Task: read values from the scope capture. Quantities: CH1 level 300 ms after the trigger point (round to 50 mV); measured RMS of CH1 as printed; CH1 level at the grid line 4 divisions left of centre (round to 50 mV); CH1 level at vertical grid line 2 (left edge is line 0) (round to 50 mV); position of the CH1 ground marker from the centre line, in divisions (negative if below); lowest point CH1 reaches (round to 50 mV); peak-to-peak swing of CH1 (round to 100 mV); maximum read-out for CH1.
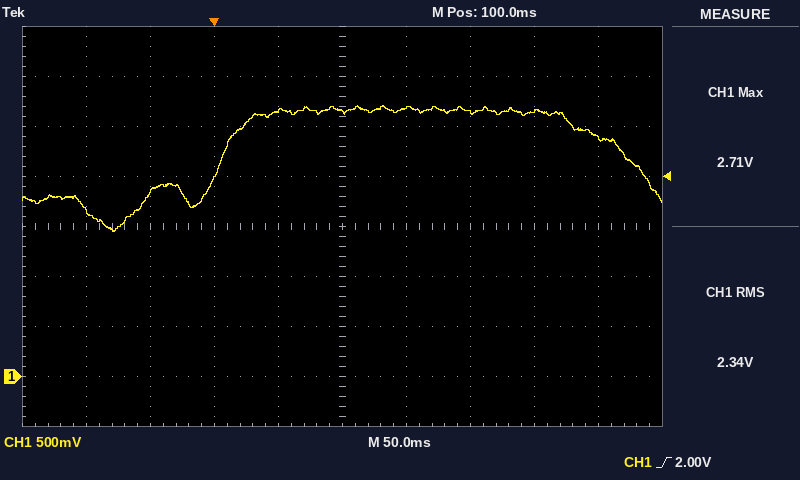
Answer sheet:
2.40 V
2.34 V
1.65 V
1.85 V
-3.0 div
1.45 V
1.30 V
2.71 V
